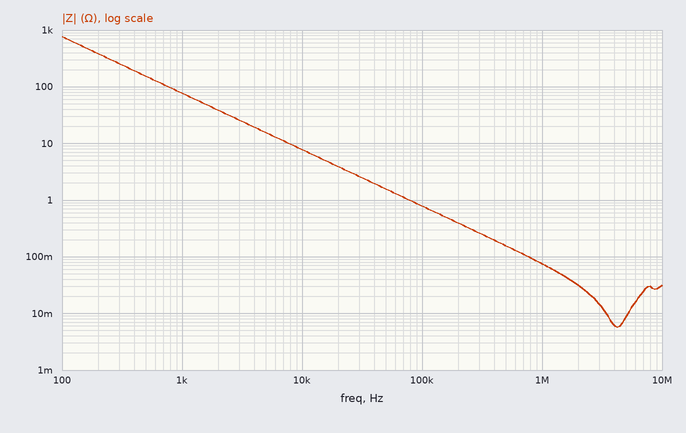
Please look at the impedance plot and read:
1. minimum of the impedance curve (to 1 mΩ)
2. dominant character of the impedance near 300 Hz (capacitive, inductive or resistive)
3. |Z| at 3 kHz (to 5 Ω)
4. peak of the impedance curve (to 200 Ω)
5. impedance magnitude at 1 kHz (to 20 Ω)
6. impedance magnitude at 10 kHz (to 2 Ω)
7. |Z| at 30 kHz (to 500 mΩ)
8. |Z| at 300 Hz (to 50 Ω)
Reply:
6 mΩ
capacitive
25 Ω
800 Ω
80 Ω
8 Ω
2.5 Ω
250 Ω
